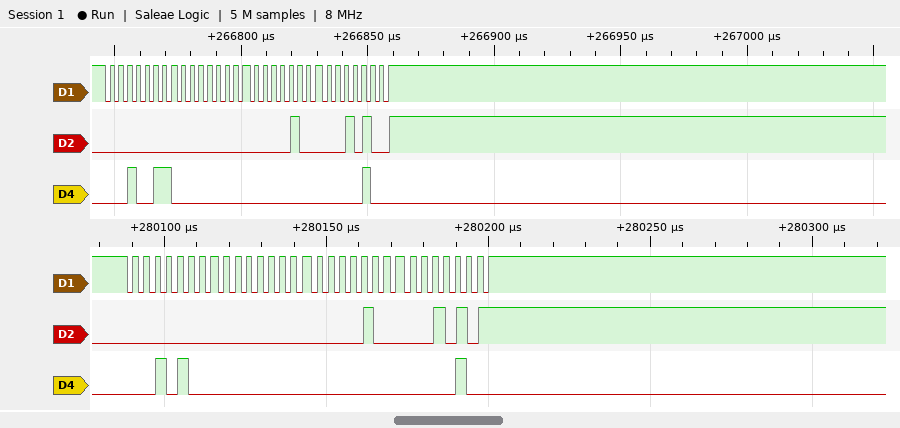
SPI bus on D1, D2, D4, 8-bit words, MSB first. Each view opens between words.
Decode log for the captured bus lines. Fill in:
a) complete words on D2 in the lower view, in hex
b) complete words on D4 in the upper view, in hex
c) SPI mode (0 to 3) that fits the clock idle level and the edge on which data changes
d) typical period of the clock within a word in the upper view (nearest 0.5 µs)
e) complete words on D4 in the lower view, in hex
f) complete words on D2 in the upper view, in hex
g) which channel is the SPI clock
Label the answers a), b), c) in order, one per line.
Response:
a) 00, 00, 04, 15
b) 13, 00, 00, 04
c) 2
d) 3.5 µs
e) 14, 00, 00, 04
f) 00, 00, 04, 14
g) D1
